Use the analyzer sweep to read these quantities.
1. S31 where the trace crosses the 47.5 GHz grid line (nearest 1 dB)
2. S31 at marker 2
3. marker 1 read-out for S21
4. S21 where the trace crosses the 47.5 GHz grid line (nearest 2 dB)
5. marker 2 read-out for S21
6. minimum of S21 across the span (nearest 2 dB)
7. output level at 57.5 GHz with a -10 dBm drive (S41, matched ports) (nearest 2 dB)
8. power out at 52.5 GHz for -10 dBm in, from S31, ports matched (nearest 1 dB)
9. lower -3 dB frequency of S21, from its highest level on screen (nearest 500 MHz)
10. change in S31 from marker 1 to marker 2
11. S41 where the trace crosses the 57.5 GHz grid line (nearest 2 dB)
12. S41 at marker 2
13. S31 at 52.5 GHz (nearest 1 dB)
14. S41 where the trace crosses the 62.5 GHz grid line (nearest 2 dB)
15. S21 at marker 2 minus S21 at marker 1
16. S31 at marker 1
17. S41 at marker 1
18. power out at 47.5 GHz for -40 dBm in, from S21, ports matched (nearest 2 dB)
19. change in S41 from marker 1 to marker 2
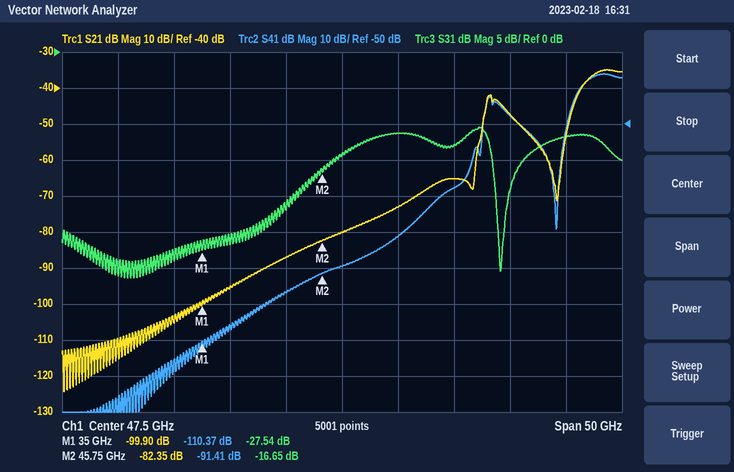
-14 dB
-16.65 dB
-99.90 dB
-80 dB
-82.35 dB
-124 dB
-78 dBm
-21 dBm
69.5 GHz
10.89 dB
-68 dB
-91.41 dB
-11 dB
-48 dB
17.55 dB
-27.54 dB
-110.37 dB
-120 dBm
18.96 dB
